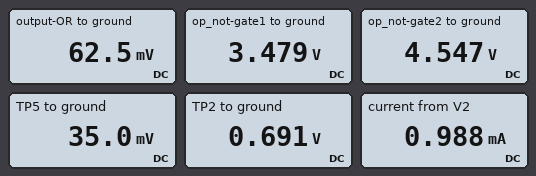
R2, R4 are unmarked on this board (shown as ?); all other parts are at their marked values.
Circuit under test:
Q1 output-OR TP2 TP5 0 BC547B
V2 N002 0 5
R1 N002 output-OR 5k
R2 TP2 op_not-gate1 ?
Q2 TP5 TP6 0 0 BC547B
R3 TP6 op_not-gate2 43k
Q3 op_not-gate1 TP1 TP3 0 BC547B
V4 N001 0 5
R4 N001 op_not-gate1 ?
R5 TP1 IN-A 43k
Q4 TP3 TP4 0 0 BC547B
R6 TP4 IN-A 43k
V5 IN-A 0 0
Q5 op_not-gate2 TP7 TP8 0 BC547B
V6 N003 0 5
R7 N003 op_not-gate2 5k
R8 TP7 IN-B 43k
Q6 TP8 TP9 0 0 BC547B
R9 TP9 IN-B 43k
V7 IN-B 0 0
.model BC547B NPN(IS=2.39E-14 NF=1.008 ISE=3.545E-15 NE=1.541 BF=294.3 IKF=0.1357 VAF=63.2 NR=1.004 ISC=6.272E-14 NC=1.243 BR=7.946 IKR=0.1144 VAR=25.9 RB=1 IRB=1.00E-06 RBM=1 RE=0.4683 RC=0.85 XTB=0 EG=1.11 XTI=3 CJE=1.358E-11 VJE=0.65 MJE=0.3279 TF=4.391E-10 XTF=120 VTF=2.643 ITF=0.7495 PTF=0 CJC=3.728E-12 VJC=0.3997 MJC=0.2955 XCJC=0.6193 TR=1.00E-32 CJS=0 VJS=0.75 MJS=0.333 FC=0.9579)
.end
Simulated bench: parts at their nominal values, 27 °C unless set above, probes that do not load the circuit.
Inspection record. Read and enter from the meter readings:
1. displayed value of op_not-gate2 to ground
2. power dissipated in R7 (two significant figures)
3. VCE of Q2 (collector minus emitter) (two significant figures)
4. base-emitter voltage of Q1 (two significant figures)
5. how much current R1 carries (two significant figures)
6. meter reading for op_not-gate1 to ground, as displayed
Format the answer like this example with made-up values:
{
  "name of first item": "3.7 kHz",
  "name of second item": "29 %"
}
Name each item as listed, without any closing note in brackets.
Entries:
{
  "displayed value of op_not-gate2 to ground": "4.547 V",
  "power dissipated in R7": "41 µW",
  "VCE of Q2 (collector minus emitter)": "35 mV",
  "base-emitter voltage of Q1": "660 mV",
  "how much current R1 carries": "990 µA",
  "meter reading for op_not-gate1 to ground, as displayed": "3.479 V"
}
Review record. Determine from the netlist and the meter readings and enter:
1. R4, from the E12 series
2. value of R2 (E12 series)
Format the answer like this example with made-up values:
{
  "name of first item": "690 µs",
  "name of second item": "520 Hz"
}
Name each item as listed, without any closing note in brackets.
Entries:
{
  "R4, from the E12 series": "12 kΩ",
  "value of R2": "22 kΩ"
}
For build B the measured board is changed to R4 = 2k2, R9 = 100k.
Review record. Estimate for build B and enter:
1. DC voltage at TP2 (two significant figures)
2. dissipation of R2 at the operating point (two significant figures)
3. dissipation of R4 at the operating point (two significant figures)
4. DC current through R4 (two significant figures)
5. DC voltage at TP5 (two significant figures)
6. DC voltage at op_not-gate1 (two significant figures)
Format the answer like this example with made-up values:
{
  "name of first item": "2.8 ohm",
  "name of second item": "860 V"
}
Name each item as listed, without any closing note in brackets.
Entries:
{
  "DC voltage at TP2": "700 mV",
  "dissipation of R2 at the operating point": "700 µW",
  "dissipation of R4 at the operating point": "70 µW",
  "DC current through R4": "180 µA",
  "DC voltage at TP5": "36 mV",
  "DC voltage at op_not-gate1": "4.6 V"
}
